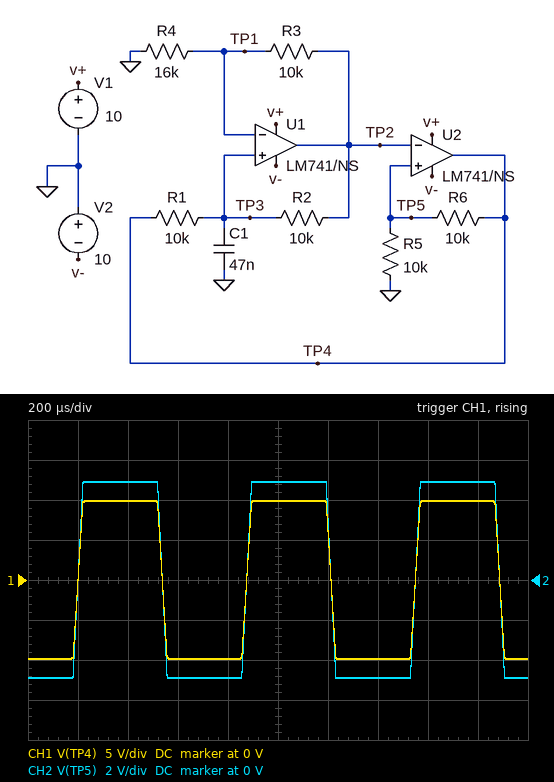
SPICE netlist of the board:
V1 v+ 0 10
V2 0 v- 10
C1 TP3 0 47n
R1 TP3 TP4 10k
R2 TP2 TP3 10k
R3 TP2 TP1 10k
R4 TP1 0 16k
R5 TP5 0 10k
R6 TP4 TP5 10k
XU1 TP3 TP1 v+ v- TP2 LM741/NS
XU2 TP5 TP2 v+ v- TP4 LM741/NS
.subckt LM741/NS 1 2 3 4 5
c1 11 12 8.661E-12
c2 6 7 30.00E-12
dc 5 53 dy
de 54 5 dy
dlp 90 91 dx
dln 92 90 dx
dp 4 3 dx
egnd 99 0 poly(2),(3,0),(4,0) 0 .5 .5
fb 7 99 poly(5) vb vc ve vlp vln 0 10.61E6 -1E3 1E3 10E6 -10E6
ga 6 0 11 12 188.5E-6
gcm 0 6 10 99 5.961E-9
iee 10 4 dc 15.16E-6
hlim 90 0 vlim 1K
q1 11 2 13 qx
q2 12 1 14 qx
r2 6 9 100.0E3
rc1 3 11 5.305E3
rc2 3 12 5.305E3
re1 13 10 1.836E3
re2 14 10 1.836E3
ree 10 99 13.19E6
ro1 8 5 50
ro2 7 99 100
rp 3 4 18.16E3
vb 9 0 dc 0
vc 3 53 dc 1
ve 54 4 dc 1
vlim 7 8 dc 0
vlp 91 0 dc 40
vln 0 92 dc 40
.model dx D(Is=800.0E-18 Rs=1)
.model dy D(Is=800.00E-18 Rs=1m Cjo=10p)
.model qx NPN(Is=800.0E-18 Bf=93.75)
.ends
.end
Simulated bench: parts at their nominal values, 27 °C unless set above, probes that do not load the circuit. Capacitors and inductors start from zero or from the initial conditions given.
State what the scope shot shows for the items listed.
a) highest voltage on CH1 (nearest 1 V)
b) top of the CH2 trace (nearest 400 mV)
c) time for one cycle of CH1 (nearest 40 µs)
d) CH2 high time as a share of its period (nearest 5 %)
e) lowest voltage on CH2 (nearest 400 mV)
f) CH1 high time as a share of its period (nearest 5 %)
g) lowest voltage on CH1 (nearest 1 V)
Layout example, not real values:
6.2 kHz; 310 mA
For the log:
10 V; 4.8 V; 680 µs; 50 %; -4.8 V; 50 %; -10 V
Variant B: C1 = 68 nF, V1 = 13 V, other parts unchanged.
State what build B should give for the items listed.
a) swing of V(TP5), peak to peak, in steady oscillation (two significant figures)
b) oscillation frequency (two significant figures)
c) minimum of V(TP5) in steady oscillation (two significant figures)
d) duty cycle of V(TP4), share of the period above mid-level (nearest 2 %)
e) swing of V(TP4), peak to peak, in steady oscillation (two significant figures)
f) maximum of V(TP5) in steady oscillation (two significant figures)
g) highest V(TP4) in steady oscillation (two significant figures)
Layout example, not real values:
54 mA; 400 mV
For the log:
11 V; 1.0 kHz; -4.9 V; 44 %; 23 V; 6.4 V; 13 V
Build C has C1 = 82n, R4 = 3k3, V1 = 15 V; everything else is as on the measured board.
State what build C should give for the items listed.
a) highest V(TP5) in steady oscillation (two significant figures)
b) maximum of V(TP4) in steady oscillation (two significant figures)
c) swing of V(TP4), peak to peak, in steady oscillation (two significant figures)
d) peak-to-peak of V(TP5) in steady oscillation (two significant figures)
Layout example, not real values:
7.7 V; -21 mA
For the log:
7.4 V; 15 V; 25 V; 12 V
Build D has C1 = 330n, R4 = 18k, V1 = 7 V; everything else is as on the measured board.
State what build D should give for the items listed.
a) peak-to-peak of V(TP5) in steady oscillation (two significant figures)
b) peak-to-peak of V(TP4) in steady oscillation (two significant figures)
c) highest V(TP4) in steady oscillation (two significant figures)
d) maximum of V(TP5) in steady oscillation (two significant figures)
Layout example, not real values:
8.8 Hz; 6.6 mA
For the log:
8.3 V; 17 V; 6.8 V; 3.4 V
